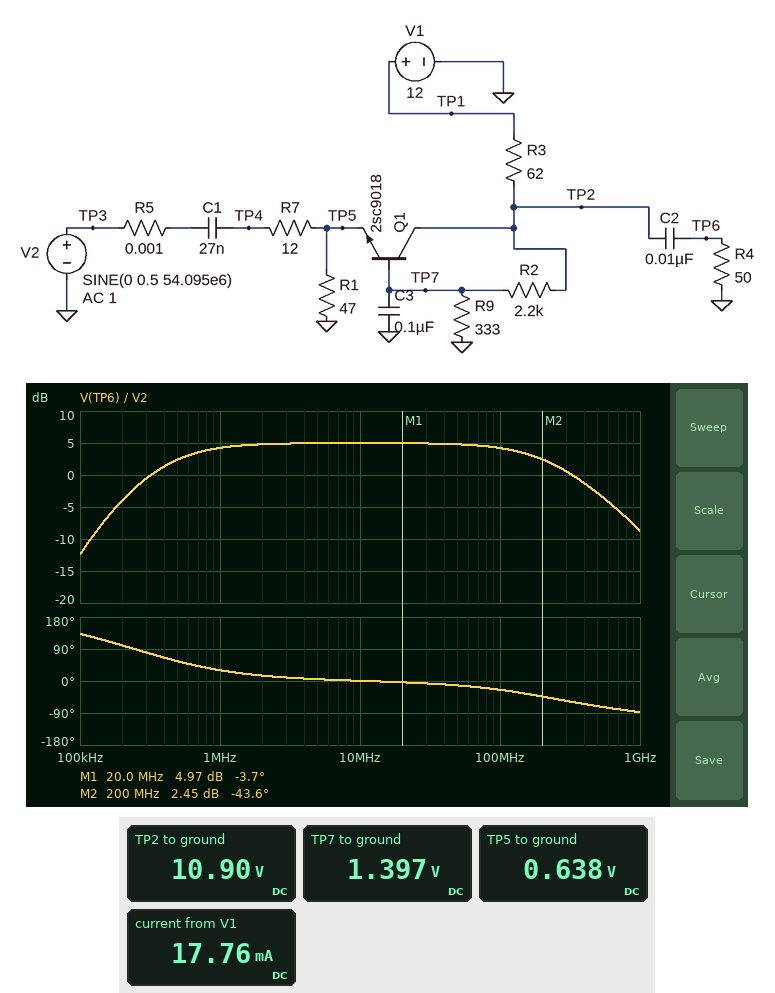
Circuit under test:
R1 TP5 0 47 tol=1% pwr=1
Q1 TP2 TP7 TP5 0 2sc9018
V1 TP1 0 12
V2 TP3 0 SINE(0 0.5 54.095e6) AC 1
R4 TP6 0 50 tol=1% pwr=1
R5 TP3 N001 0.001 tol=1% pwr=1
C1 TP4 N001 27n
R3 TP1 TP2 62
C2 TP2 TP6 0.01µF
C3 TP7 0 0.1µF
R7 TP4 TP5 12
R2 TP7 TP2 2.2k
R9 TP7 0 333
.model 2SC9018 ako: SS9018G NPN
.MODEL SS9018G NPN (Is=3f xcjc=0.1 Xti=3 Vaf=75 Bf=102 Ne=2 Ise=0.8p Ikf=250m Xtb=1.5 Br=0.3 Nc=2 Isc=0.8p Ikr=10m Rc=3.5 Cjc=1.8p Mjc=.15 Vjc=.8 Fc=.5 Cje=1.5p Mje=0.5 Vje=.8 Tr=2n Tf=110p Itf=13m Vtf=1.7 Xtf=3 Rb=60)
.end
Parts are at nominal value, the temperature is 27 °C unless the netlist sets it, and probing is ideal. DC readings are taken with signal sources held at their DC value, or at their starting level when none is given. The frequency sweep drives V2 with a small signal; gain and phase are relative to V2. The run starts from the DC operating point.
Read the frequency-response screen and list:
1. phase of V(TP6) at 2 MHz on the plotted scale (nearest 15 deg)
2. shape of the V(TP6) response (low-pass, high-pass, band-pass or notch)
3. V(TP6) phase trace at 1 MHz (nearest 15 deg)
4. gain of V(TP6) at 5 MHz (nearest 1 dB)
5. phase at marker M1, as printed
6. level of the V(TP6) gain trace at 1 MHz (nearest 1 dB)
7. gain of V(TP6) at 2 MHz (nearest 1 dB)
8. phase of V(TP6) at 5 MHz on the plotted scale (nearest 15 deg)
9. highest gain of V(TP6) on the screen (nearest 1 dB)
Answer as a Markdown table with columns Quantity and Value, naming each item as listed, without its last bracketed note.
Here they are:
| Quantity | Value |
|---|---|
| phase of V(TP6) at 2 MHz on the plotted scale | 15 deg |
| shape of the V(TP6) response | band-pass |
| V(TP6) phase trace at 1 MHz | 30 deg |
| gain of V(TP6) at 5 MHz | 5 dB |
| phase at marker M1, as printed | -3.7 deg |
| level of the V(TP6) gain trace at 1 MHz | 4 dB |
| gain of V(TP6) at 2 MHz | 5 dB |
| phase of V(TP6) at 5 MHz on the plotted scale | 0 deg |
| highest gain of V(TP6) on the screen | 5 dB |
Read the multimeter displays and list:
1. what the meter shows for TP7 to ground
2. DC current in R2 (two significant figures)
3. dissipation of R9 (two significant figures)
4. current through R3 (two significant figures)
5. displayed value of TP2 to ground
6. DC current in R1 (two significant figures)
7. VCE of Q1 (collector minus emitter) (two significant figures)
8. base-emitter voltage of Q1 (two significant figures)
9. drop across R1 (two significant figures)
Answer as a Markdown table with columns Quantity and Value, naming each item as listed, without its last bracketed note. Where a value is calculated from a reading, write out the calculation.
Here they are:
| Quantity | Value |
|---|---|
| what the meter shows for TP7 to ground | 1.397 V |
| DC current in R2 | (10.9 V - 1.397 V) / 2.2 kΩ = 4.3 mA |
| dissipation of R9 | (1.397 V)^2 / 333 Ω = 5.9 mW |
| current through R3 | (12 V - 10.9 V) / 62 Ω = 18 mA |
| displayed value of TP2 to ground | 10.90 V |
| DC current in R1 | (638 mV) / 47 Ω = 14 mA |
| VCE of Q1 (collector minus emitter) | 10.9 V - 638 mV = 10 V |
| base-emitter voltage of Q1 | 1.397 V - 638 mV = 760 mV |
| drop across R1 | 638 mV = 640 mV |
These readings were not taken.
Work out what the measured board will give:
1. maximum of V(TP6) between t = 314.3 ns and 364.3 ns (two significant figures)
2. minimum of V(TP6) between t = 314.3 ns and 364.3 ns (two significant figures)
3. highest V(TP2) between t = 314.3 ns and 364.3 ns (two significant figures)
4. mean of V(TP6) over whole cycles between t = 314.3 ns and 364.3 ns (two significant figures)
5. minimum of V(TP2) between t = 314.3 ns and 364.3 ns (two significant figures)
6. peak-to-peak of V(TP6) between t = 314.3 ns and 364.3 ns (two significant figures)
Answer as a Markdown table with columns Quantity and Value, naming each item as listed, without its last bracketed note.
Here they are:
| Quantity | Value |
|---|---|
| maximum of V(TP6) between t = 314.3 ns and 364.3 ns | 400 mV |
| minimum of V(TP6) between t = 314.3 ns and 364.3 ns | -820 mV |
| highest V(TP2) between t = 314.3 ns and 364.3 ns | 11 V |
| mean of V(TP6) over whole cycles between t = 314.3 ns and 364.3 ns | -69 mV |
| minimum of V(TP2) between t = 314.3 ns and 364.3 ns | 10 V |
| peak-to-peak of V(TP6) between t = 314.3 ns and 364.3 ns | 1.2 V |
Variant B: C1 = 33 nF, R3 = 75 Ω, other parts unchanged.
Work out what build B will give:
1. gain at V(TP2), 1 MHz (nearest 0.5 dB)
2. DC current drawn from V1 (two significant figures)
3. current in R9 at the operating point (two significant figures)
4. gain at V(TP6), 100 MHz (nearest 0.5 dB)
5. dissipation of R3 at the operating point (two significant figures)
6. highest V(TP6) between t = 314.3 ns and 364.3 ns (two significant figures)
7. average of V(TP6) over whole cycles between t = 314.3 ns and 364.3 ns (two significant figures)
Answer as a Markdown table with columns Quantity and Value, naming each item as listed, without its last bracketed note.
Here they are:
| Quantity | Value |
|---|---|
| gain at V(TP2), 1 MHz | 5.5 dB |
| DC current drawn from V1 | 17 mA |
| current in R9 at the operating point | 4.1 mA |
| gain at V(TP6), 100 MHz | 5.0 dB |
| dissipation of R3 at the operating point | 22 mW |
| highest V(TP6) between t = 314.3 ns and 364.3 ns | 420 mV |
| average of V(TP6) over whole cycles between t = 314.3 ns and 364.3 ns | -86 mV |
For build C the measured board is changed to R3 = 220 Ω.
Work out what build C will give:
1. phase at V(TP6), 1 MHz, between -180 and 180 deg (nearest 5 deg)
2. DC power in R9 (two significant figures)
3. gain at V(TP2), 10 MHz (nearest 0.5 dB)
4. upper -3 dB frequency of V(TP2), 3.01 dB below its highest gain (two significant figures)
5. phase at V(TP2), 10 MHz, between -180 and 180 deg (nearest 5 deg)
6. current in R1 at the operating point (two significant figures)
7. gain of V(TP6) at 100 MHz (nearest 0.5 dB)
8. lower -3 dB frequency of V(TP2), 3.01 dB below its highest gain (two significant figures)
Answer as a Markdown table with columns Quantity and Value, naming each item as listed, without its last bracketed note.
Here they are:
| Quantity | Value |
|---|---|
| phase at V(TP6), 1 MHz, between -180 and 180 deg | 25 deg |
| DC power in R9 | 4.2 mW |
| gain at V(TP2), 10 MHz | 7.5 dB |
| upper -3 dB frequency of V(TP2), 3.01 dB below its highest gain | 230 MHz |
| phase at V(TP2), 10 MHz, between -180 and 180 deg | 0 deg |
| current in R1 at the operating point | 9.3 mA |
| gain of V(TP6) at 100 MHz | 7.0 dB |
| lower -3 dB frequency of V(TP2), 3.01 dB below its highest gain | 100 kHz |
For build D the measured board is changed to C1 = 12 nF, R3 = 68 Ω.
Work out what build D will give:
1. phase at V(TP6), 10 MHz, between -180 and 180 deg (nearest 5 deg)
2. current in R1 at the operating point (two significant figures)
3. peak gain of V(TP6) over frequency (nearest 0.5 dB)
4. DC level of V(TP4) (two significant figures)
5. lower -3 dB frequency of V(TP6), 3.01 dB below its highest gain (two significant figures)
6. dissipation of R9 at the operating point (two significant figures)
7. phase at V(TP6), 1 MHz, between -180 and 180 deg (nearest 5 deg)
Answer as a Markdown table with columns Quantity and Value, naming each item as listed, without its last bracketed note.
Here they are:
| Quantity | Value |
|---|---|
| phase at V(TP6), 10 MHz, between -180 and 180 deg | 5 deg |
| current in R1 at the operating point | 13 mA |
| peak gain of V(TP6) over frequency | 5.5 dB |
| DC level of V(TP4) | 630 mV |
| lower -3 dB frequency of V(TP6), 3.01 dB below its highest gain | 930 kHz |
| dissipation of R9 at the operating point | 5.8 mW |
| phase at V(TP6), 1 MHz, between -180 and 180 deg | 50 deg |
